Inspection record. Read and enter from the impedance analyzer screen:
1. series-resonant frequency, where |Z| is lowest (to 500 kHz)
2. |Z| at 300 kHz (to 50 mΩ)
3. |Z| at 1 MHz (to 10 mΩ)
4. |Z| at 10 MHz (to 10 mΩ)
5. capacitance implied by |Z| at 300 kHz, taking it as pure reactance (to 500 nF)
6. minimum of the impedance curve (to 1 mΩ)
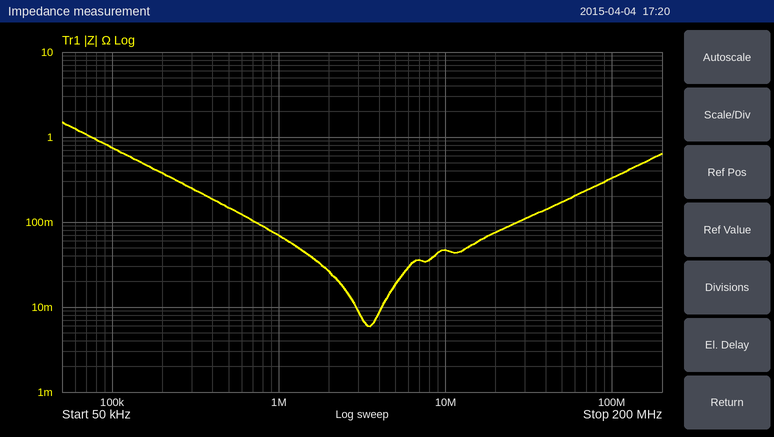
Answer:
3.5 MHz
250 mΩ
70 mΩ
50 mΩ
2.0 µF
6 mΩ
